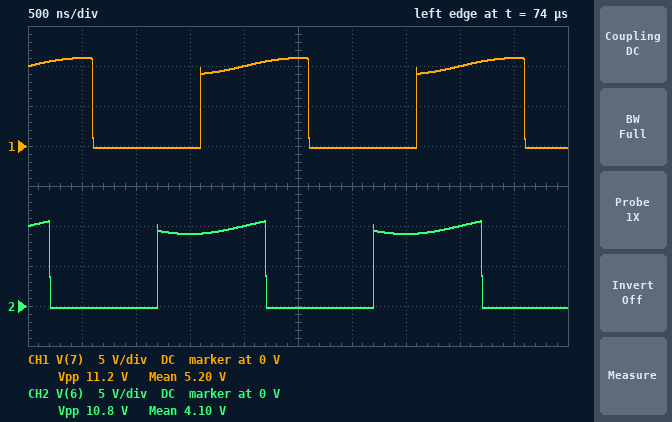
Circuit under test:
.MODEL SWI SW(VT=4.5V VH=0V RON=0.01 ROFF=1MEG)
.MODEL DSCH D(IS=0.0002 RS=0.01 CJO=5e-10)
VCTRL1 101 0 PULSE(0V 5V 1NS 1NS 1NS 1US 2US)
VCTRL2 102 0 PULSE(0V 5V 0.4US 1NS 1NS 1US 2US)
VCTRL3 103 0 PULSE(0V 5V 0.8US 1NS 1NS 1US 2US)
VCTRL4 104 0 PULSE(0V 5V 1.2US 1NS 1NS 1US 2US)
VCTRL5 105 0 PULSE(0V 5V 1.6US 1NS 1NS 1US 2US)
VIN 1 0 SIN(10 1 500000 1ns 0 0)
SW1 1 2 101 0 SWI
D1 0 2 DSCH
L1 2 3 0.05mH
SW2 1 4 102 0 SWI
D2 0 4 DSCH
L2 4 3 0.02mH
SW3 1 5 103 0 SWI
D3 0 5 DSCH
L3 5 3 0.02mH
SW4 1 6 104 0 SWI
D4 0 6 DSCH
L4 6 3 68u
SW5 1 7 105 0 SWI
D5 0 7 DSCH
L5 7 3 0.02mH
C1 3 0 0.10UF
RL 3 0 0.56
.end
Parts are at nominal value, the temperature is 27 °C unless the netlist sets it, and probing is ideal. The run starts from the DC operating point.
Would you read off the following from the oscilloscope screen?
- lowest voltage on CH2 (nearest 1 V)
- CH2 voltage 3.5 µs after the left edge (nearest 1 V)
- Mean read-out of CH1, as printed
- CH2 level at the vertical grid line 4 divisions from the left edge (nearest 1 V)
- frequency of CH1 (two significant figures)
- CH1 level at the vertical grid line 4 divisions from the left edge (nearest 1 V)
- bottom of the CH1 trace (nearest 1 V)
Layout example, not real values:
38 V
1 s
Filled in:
0 V
9 V
5.20 V
10 V
500 kHz
10 V
0 V
